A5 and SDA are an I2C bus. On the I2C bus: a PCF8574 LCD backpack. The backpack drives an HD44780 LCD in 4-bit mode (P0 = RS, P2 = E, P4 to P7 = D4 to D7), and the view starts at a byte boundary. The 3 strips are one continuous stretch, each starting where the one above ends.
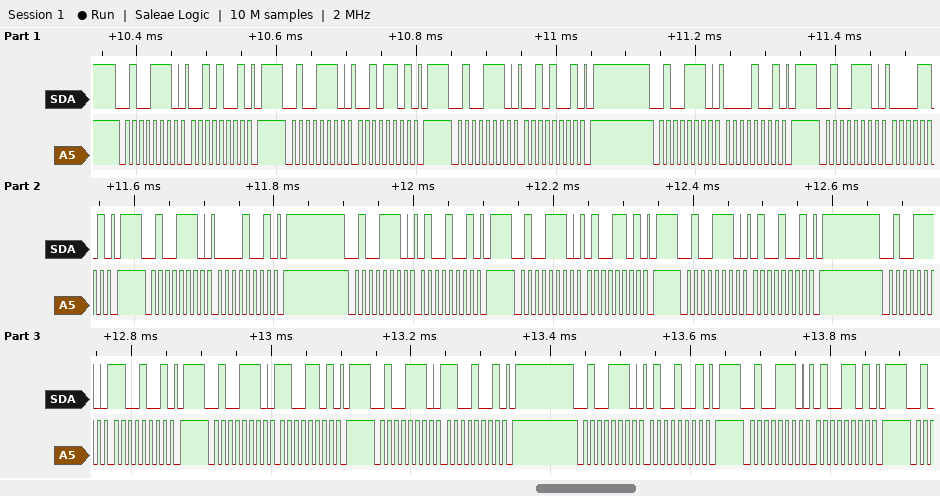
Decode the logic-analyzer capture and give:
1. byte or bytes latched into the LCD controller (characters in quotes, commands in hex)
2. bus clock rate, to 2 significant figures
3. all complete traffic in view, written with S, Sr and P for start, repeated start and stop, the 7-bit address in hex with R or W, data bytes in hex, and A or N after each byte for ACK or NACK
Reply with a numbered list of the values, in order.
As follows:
1. ' ' 'L'
2. 100 kHz
3. S 27W A 29 A P S 27W A 2D A P S 27W A 29 A P S 27W A 09 A P S 27W A 0D A P S 27W A 09 A P S 27W A 49 A P S 27W A 4D A P S 27W A 49 A P S 27W A C9 A P S 27W A CD A P S 27W A C9 A P S 27W A 49 A P S 27W A 4D A P
